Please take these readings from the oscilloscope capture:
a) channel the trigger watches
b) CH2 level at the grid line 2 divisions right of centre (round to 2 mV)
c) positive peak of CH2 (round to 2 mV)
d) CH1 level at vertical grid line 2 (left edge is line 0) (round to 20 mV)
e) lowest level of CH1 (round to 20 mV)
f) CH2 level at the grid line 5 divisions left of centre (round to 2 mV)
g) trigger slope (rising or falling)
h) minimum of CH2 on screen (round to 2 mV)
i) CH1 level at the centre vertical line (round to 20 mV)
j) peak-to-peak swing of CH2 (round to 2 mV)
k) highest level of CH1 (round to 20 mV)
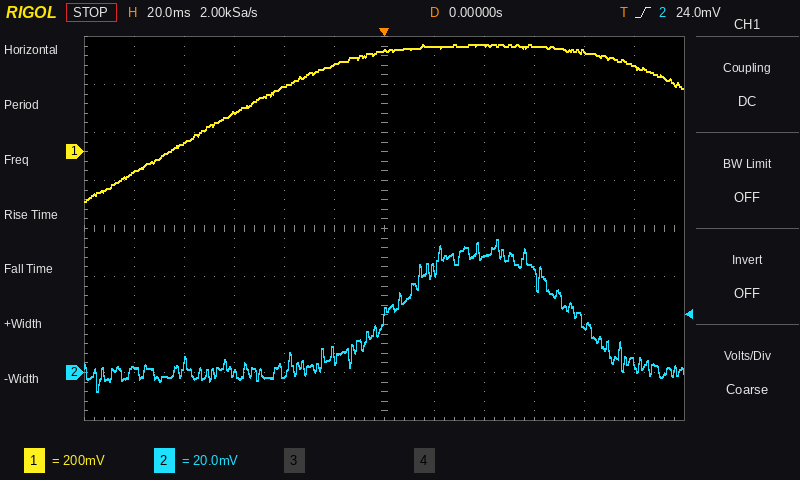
CH2
48 mV
56 mV
40 mV
-200 mV
2 mV
rising
-8 mV
420 mV
64 mV
440 mV
